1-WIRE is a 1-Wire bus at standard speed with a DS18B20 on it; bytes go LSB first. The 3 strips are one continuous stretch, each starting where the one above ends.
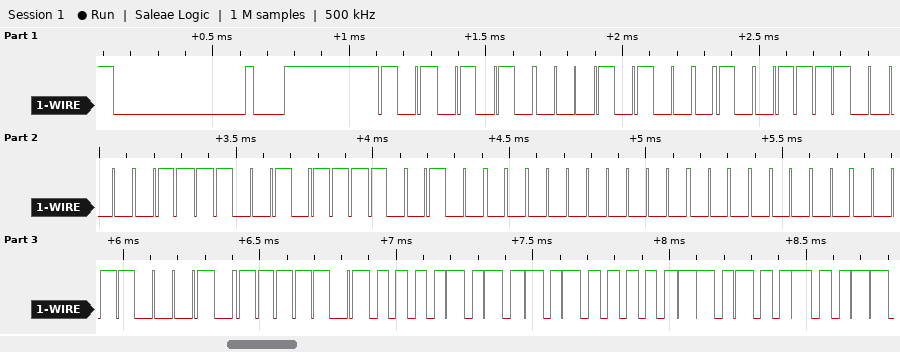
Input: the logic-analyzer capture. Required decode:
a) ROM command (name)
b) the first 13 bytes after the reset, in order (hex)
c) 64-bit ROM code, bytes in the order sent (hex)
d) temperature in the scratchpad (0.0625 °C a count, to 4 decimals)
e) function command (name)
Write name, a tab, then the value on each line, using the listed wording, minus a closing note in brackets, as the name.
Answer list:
ROM command	Match ROM
the first 13 bytes after the reset, in order	55 28 F2 E0 E9 09 00 00 8C BE 50 05 4B
64-bit ROM code, bytes in the order sent	28 F2 E0 E9 09 00 00 8C
temperature in the scratchpad	85.0000 °C
function command	Read Scratchpad
